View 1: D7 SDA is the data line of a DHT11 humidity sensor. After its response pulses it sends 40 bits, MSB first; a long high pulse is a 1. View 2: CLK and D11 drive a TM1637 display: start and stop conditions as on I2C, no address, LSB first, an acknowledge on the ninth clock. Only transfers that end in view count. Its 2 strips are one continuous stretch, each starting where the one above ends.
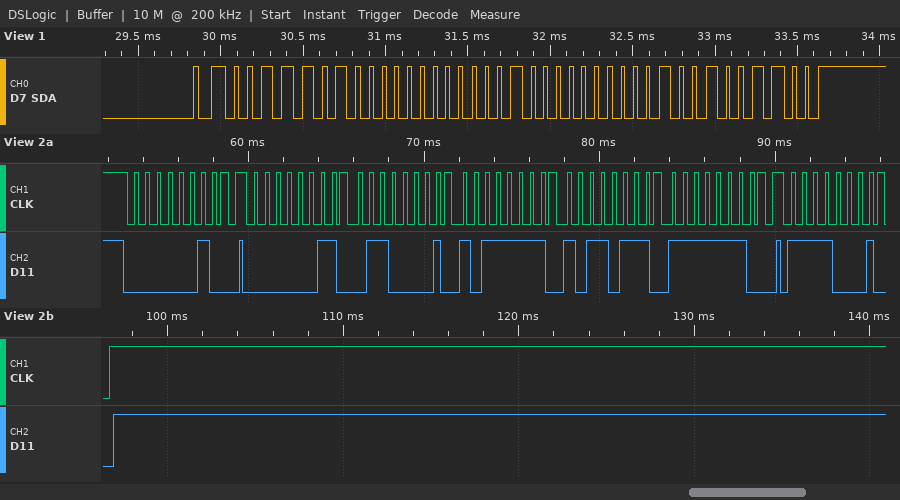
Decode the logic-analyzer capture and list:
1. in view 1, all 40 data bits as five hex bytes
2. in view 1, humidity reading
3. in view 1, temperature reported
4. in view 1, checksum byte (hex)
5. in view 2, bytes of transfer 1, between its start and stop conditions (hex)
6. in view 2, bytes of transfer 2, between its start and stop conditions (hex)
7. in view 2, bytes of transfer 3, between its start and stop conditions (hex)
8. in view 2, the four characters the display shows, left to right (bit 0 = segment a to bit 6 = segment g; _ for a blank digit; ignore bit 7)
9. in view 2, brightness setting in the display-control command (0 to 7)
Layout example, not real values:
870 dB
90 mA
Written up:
3A 00 10 02 4C
58 %
16.2 °C
0x4C
40
C0 86 FD ED 7F
8F
1658
7
